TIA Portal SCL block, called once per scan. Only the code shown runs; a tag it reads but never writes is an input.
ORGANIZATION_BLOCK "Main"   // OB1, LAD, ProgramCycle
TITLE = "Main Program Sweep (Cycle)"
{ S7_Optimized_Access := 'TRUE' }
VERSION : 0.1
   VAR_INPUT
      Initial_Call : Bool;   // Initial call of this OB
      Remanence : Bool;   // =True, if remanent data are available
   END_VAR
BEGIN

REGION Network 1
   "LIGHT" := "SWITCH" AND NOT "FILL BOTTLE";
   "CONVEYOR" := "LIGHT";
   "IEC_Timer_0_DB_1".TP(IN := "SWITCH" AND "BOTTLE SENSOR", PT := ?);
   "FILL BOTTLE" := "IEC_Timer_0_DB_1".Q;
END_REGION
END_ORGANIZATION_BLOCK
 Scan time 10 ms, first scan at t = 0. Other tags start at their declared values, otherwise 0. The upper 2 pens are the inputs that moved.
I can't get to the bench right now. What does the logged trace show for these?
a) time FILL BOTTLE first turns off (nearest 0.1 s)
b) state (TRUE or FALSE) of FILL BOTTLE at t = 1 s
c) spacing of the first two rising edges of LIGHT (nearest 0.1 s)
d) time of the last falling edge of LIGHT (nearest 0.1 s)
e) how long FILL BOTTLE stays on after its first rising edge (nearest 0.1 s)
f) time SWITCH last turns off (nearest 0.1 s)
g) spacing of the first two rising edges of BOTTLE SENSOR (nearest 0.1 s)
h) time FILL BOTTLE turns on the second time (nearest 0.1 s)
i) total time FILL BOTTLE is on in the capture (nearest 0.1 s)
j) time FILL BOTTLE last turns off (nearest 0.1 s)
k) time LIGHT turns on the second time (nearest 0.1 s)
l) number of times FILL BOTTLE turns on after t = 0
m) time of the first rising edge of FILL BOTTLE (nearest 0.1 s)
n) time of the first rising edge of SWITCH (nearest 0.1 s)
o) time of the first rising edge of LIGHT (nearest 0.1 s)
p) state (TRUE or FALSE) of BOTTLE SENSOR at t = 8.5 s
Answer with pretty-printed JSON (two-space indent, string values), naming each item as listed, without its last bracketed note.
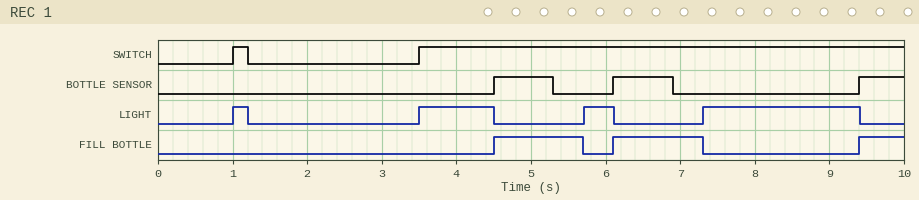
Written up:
{
  "time FILL BOTTLE first turns off": "5.7 s",
  "state (TRUE or FALSE) of FILL BOTTLE at t = 1 s": "FALSE",
  "spacing of the first two rising edges of LIGHT": "2.5 s",
  "time of the last falling edge of LIGHT": "9.4 s",
  "how long FILL BOTTLE stays on after its first rising edge": "1.2 s",
  "time SWITCH last turns off": "1.2 s",
  "spacing of the first two rising edges of BOTTLE SENSOR": "1.6 s",
  "time FILL BOTTLE turns on the second time": "6.1 s",
  "total time FILL BOTTLE is on in the capture": "3.0 s",
  "time FILL BOTTLE last turns off": "7.3 s",
  "time LIGHT turns on the second time": "3.5 s",
  "number of times FILL BOTTLE turns on after t = 0": "3",
  "time of the first rising edge of FILL BOTTLE": "4.5 s",
  "time of the first rising edge of SWITCH": "1.0 s",
  "time of the first rising edge of LIGHT": "1.0 s",
  "state (TRUE or FALSE) of BOTTLE SENSOR at t = 8.5 s": "FALSE"
}
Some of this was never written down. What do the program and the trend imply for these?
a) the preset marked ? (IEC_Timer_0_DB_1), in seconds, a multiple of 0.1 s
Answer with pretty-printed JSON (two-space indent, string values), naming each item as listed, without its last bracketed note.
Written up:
{
  "the preset marked ? (IEC_Timer_0_DB_1), in seconds, a multiple of 0.1 s": "1.2 s"
}
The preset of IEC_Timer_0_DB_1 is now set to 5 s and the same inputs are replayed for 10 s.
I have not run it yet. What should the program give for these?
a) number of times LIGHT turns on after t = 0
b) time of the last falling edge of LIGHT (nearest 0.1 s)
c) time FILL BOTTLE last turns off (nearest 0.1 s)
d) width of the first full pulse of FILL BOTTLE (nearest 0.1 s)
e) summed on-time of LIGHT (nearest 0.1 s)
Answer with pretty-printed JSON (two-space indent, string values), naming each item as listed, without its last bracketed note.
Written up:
{
  "number of times LIGHT turns on after t = 0": "3",
  "time of the last falling edge of LIGHT": "4.5 s",
  "time FILL BOTTLE last turns off": "9.5 s",
  "width of the first full pulse of FILL BOTTLE": "5.0 s",
  "summed on-time of LIGHT": "1.7 s"
}
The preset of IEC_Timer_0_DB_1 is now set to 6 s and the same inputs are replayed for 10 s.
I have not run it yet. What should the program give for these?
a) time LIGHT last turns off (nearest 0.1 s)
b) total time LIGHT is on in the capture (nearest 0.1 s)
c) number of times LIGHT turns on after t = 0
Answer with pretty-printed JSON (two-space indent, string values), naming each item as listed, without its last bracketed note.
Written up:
{
  "time LIGHT last turns off": "4.5 s",
  "total time LIGHT is on in the capture": "1.2 s",
  "number of times LIGHT turns on after t = 0": "2"
}
